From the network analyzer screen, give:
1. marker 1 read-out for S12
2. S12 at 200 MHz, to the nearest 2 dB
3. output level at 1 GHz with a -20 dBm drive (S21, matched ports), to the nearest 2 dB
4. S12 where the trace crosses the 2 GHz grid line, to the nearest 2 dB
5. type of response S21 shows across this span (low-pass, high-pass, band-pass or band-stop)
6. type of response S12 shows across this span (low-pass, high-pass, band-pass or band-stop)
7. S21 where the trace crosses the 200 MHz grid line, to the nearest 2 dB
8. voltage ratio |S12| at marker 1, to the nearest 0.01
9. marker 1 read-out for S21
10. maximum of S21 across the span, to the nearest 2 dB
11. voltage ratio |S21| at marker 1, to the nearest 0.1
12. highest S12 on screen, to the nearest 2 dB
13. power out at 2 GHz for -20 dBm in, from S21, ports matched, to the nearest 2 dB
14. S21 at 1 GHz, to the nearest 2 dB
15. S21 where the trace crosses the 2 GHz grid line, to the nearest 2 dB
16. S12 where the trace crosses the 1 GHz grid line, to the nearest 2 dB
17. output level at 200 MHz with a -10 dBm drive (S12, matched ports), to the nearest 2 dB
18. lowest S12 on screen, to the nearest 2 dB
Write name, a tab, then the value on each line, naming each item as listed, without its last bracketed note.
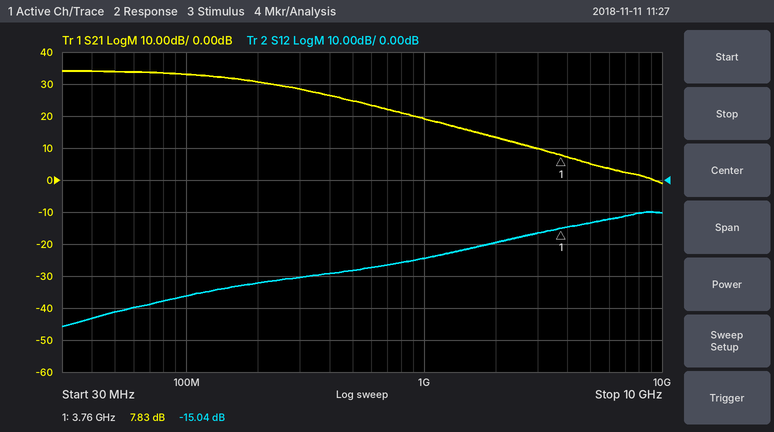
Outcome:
marker 1 read-out for S12	-15.04 dB
S12 at 200 MHz, to the nearest 2 dB	-32 dB
output level at 1 GHz with a -20 dBm drive (S21, matched ports), to the nearest 2 dB	0 dBm
S12 where the trace crosses the 2 GHz grid line, to the nearest 2 dB	-20 dB
type of response S21 shows across this span	low-pass
type of response S12 shows across this span	high-pass
S21 where the trace crosses the 200 MHz grid line, to the nearest 2 dB	30 dB
voltage ratio |S12| at marker 1, to the nearest 0.01	0.18
marker 1 read-out for S21	7.83 dB
maximum of S21 across the span, to the nearest 2 dB	34 dB
voltage ratio |S21| at marker 1, to the nearest 0.1	2.5
highest S12 on screen, to the nearest 2 dB	-10 dB
power out at 2 GHz for -20 dBm in, from S21, ports matched, to the nearest 2 dB	-6 dBm
S21 at 1 GHz, to the nearest 2 dB	20 dB
S21 where the trace crosses the 2 GHz grid line, to the nearest 2 dB	14 dB
S12 where the trace crosses the 1 GHz grid line, to the nearest 2 dB	-24 dB
output level at 200 MHz with a -10 dBm drive (S12, matched ports), to the nearest 2 dB	-42 dBm
lowest S12 on screen, to the nearest 2 dB	-46 dB
